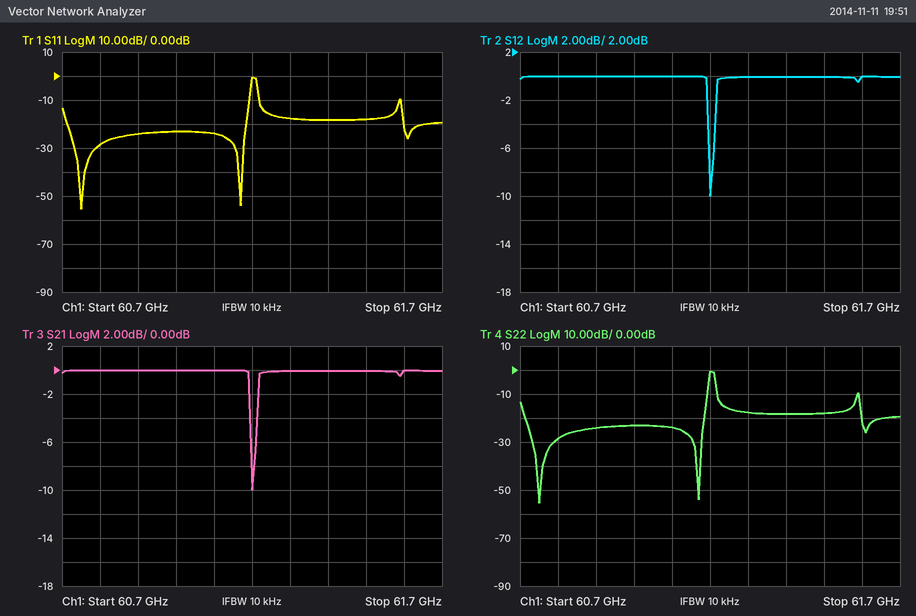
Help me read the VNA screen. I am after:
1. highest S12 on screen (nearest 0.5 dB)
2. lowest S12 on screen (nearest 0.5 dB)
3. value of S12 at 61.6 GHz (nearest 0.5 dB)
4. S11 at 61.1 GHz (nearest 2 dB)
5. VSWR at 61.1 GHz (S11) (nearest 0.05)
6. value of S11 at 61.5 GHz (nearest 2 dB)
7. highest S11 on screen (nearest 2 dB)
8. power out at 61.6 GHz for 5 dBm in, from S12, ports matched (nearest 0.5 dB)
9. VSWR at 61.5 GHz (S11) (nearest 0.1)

0.0 dB
-10.0 dB
0.0 dB
-24 dB
1.15
-18 dB
0 dB
5.0 dBm
1.3
